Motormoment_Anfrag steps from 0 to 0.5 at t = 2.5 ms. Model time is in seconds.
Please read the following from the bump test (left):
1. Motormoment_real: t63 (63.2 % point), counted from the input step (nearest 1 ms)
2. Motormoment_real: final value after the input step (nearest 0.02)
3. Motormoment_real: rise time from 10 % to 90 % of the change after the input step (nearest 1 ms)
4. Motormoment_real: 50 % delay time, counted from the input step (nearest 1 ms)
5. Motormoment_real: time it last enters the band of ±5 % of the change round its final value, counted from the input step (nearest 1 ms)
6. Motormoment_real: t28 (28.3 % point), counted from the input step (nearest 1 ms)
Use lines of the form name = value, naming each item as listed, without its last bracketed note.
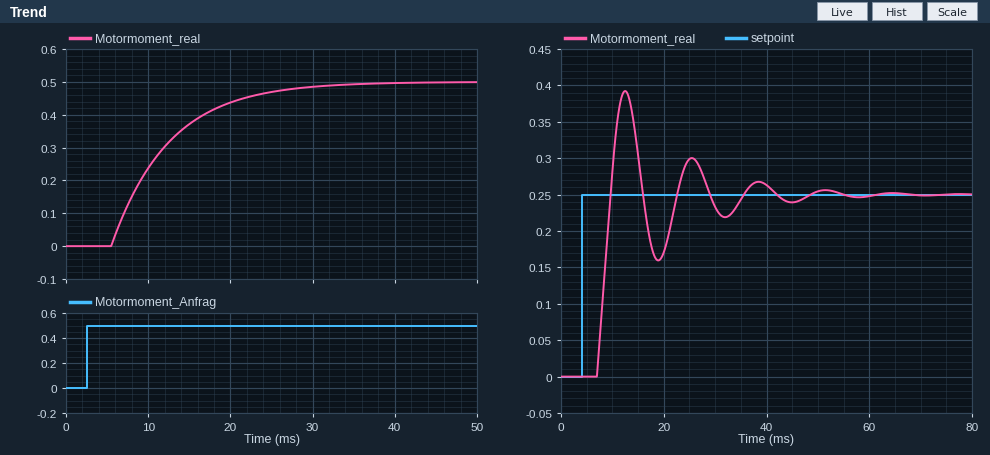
Motormoment_real: t63 (63.2 % point), counted from the input step = 10 ms
Motormoment_real: final value after the input step = 0.50
Motormoment_real: rise time from 10 % to 90 % of the change after the input step = 15 ms
Motormoment_real: 50 % delay time, counted from the input step = 8 ms
Motormoment_real: time it last enters the band of ±5 % of the change round its final value, counted from the input step = 24 ms
Motormoment_real: t28 (28.3 % point), counted from the input step = 5 ms
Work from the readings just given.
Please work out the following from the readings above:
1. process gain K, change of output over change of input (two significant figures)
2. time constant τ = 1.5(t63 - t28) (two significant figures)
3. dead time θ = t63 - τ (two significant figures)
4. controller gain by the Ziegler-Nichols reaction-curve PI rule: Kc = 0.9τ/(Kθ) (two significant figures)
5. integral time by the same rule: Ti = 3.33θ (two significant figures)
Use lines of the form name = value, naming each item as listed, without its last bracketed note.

process gain K, change of output over change of input = 1.0
time constant τ = 1.5(t63 - t28) = 7.5 ms
dead time θ = t63 - τ = 2.5 ms
controller gain by the Ziegler-Nichols reaction-curve PI rule: Kc = 0.9τ/(Kθ) = 2.7
integral time by the same rule: Ti = 3.33θ = 8.3 ms
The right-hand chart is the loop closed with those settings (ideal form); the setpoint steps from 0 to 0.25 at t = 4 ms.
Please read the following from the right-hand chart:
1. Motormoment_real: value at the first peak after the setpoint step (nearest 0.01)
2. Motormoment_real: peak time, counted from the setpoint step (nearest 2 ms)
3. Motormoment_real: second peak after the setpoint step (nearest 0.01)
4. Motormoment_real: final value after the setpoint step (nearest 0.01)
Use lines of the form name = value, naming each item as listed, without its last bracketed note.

Motormoment_real: value at the first peak after the setpoint step = 0.39
Motormoment_real: peak time, counted from the setpoint step = 8 ms
Motormoment_real: second peak after the setpoint step = 0.30
Motormoment_real: final value after the setpoint step = 0.25
